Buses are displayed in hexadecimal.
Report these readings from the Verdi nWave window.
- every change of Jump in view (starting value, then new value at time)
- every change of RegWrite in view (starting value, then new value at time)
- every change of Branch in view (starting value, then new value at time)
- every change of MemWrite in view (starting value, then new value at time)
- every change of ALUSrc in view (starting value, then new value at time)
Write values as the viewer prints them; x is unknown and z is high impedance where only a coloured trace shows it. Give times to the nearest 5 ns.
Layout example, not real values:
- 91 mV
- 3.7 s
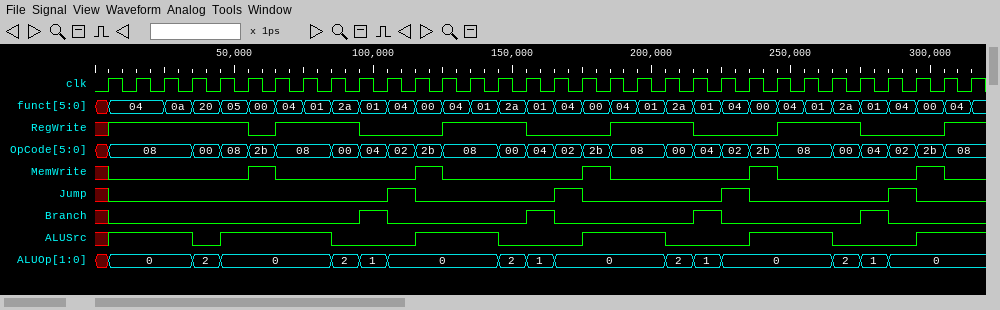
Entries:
- x, 0 at 5 ns, 1 at 105 ns, 0 at 115 ns, 1 at 165 ns, 0 at 175 ns, 1 at 225 ns, 0 at 235 ns, 1 at 285 ns, 0 at 295 ns
- x, 1 at 5 ns, 0 at 55 ns, 1 at 65 ns, 0 at 95 ns, 1 at 125 ns, 0 at 155 ns, 1 at 185 ns, 0 at 215 ns, 1 at 245 ns, 0 at 275 ns, 1 at 305 ns
- x, 0 at 5 ns, 1 at 95 ns, 0 at 105 ns, 1 at 155 ns, 0 at 165 ns, 1 at 215 ns, 0 at 225 ns, 1 at 275 ns, 0 at 285 ns
- x, 0 at 5 ns, 1 at 55 ns, 0 at 65 ns, 1 at 115 ns, 0 at 125 ns, 1 at 175 ns, 0 at 185 ns, 1 at 235 ns, 0 at 245 ns, 1 at 295 ns, 0 at 305 ns
- x, 1 at 5 ns, 0 at 35 ns, 1 at 45 ns, 0 at 85 ns, 1 at 115 ns, 0 at 145 ns, 1 at 175 ns, 0 at 205 ns, 1 at 235 ns, 0 at 265 ns, 1 at 295 ns
